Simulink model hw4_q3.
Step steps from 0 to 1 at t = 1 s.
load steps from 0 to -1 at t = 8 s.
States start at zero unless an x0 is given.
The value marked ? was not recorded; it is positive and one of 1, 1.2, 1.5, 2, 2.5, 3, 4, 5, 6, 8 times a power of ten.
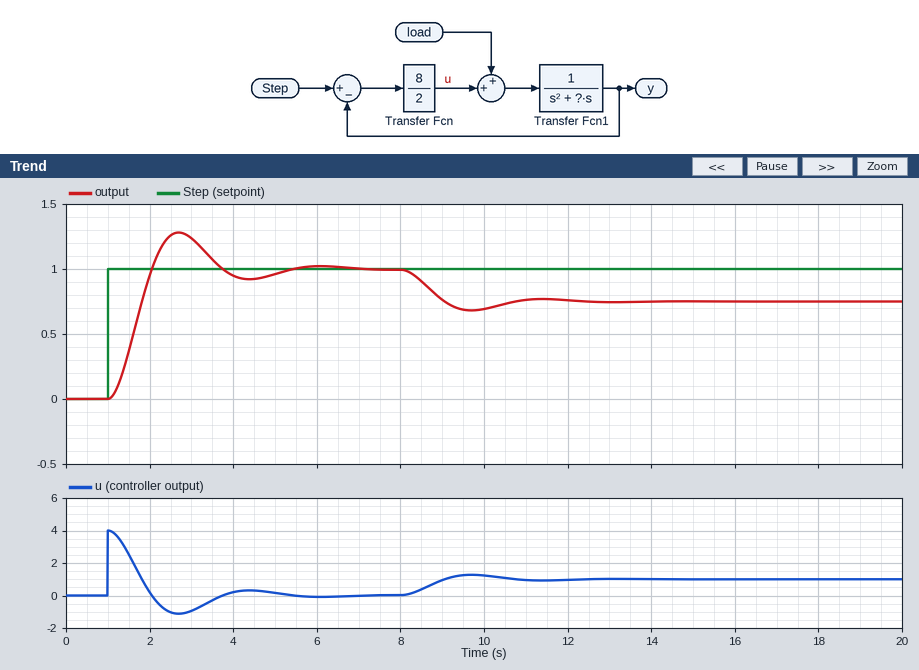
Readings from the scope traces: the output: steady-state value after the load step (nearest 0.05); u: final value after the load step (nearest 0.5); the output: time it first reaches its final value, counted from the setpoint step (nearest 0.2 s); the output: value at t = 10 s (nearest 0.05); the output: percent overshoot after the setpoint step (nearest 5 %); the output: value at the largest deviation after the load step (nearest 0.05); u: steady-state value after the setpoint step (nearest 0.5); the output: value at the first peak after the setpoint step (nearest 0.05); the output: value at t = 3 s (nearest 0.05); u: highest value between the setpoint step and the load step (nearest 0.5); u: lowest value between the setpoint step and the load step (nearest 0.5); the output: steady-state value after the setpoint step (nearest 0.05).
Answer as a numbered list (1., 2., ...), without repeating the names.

1. 0.75
2. 1.0
3. 1.0 s
4. 0.70
5. 30 %
6. 0.70
7. 0.0
8. 1.30
9. 1.25
10. 4.0
11. -1.0
12. 1.00
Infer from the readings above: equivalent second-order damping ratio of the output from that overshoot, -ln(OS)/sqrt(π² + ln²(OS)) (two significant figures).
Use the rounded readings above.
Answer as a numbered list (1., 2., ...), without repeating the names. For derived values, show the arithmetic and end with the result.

1. ln(0.3) = -1.204; 1.204 / sqrt(9.870 + 1.450) = 0.36
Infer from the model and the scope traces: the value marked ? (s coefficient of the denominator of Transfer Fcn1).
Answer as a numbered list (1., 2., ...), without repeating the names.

1. 1.5
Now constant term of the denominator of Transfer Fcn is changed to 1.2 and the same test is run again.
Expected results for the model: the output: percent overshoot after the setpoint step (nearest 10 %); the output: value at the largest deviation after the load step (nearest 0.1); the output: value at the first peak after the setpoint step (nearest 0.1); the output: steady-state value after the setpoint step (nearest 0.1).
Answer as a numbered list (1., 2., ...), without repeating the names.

1. 40 %
2. 0.8
3. 1.4
4. 1.0
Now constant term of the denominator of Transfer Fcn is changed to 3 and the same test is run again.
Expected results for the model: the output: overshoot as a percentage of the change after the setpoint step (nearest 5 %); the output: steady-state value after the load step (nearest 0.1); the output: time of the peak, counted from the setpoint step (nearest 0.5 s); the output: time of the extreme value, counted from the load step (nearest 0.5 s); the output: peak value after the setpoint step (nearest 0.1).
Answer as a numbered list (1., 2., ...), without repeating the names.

1. 20 %
2. 0.6
3. 2.0 s
4. 2.0 s
5. 1.2
